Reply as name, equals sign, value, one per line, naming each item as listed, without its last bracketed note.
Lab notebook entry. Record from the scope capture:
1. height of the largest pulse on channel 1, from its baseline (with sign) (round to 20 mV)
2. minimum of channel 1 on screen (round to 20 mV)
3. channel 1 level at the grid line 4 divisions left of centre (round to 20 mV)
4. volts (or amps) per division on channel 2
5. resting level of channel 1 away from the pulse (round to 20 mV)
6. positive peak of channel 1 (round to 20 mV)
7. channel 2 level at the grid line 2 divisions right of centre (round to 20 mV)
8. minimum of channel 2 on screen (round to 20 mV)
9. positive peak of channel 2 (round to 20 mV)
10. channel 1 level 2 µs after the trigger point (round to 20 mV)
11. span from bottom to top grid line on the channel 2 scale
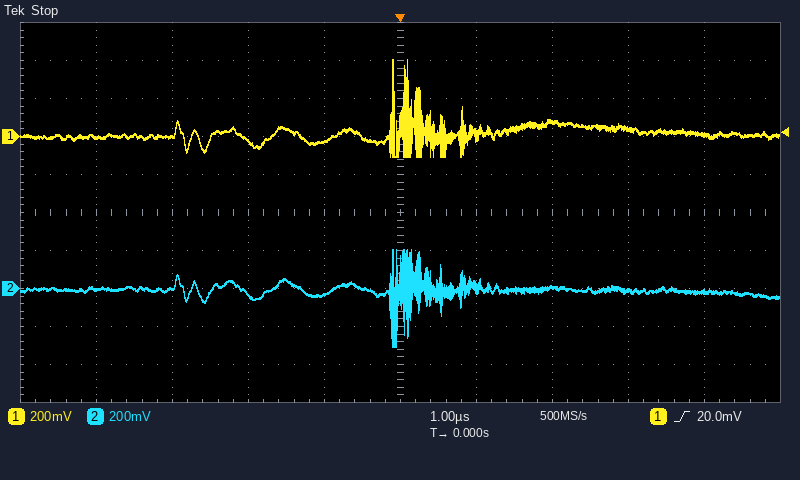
height of the largest pulse on channel 1, from its baseline (with sign) = +400 mV
minimum of channel 1 on screen = -100 mV
channel 1 level at the grid line 4 divisions left of centre = 0 mV
volts (or amps) per division on channel 2 = 200 mV
resting level of channel 1 away from the pulse = 0 mV
positive peak of channel 1 = 400 mV
channel 2 level at the grid line 2 divisions right of centre = 0 mV
minimum of channel 2 on screen = -300 mV
positive peak of channel 2 = 200 mV
channel 1 level 2 µs after the trigger point = 80 mV
span from bottom to top grid line on the channel 2 scale = 2 V
